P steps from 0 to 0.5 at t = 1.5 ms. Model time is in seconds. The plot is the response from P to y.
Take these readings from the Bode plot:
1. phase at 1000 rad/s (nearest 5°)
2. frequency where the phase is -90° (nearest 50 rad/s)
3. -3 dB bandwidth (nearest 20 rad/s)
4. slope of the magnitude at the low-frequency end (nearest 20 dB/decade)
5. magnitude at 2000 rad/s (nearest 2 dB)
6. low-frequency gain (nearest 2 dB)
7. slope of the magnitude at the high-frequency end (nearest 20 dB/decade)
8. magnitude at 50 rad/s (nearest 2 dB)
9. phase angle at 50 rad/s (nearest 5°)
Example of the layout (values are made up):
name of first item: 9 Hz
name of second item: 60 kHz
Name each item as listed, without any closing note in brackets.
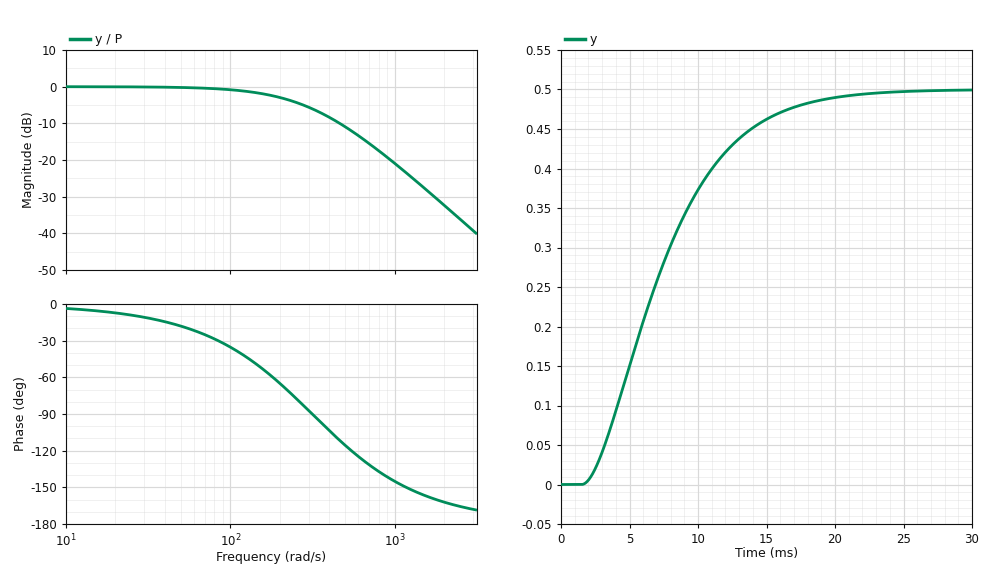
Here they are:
phase at 1000 rad/s: -145°
frequency where the phase is -90°: 300 rad/s
-3 dB bandwidth: 200 rad/s
slope of the magnitude at the low-frequency end: 0 dB/decade
magnitude at 2000 rad/s: -32 dB
low-frequency gain: 0 dB
slope of the magnitude at the high-frequency end: -40 dB/decade
magnitude at 50 rad/s: 0 dB
phase angle at 50 rad/s: -20°
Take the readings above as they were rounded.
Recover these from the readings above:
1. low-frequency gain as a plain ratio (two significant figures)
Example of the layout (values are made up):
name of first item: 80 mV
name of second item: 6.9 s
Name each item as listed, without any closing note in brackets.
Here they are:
low-frequency gain as a plain ratio: 1.0
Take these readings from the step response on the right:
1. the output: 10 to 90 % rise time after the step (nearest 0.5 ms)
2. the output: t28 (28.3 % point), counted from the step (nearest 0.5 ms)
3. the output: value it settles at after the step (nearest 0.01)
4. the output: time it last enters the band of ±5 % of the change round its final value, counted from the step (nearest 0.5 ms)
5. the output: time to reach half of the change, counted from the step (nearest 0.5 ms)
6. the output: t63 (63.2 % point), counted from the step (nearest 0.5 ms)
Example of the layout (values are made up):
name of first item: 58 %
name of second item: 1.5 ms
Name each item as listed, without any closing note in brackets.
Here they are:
the output: 10 to 90 % rise time after the step: 10.5 ms
the output: t28 (28.3 % point), counted from the step: 3.5 ms
the output: value it settles at after the step: 0.50
the output: time it last enters the band of ±5 % of the change round its final value, counted from the step: 15.0 ms
the output: time to reach half of the change, counted from the step: 5.5 ms
the output: t63 (63.2 % point), counted from the step: 7.0 ms
